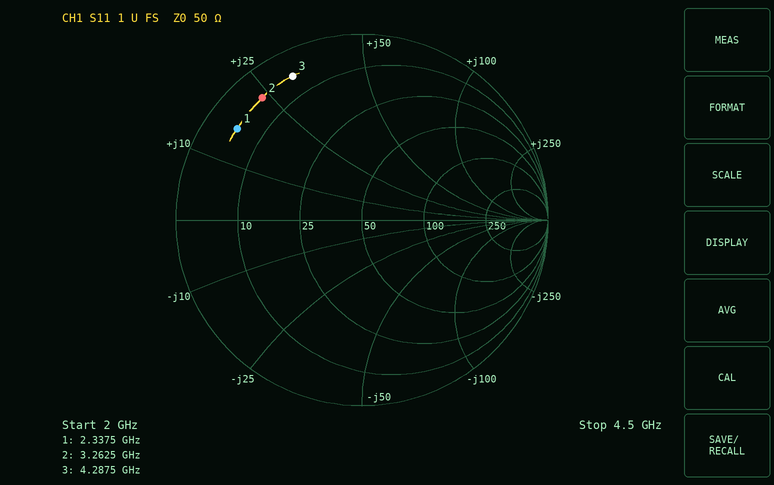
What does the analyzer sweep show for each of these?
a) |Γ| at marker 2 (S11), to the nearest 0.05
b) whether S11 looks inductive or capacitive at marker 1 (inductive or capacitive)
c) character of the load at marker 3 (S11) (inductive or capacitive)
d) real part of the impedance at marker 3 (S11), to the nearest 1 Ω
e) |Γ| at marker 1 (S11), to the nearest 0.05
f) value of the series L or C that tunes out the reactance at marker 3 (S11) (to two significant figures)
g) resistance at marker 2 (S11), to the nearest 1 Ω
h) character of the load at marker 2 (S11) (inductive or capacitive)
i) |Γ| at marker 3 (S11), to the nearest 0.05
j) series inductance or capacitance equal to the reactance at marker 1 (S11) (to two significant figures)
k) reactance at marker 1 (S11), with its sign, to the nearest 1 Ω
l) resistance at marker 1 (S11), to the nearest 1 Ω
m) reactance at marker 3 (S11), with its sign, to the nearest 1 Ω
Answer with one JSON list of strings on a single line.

["0.85", "inductive", "inductive", "5 Ω", "0.85", "1.2 pF", "5 Ω", "inductive", "0.85", "1.1 nH", "+16 Ω", "5 Ω", "+31 Ω"]
